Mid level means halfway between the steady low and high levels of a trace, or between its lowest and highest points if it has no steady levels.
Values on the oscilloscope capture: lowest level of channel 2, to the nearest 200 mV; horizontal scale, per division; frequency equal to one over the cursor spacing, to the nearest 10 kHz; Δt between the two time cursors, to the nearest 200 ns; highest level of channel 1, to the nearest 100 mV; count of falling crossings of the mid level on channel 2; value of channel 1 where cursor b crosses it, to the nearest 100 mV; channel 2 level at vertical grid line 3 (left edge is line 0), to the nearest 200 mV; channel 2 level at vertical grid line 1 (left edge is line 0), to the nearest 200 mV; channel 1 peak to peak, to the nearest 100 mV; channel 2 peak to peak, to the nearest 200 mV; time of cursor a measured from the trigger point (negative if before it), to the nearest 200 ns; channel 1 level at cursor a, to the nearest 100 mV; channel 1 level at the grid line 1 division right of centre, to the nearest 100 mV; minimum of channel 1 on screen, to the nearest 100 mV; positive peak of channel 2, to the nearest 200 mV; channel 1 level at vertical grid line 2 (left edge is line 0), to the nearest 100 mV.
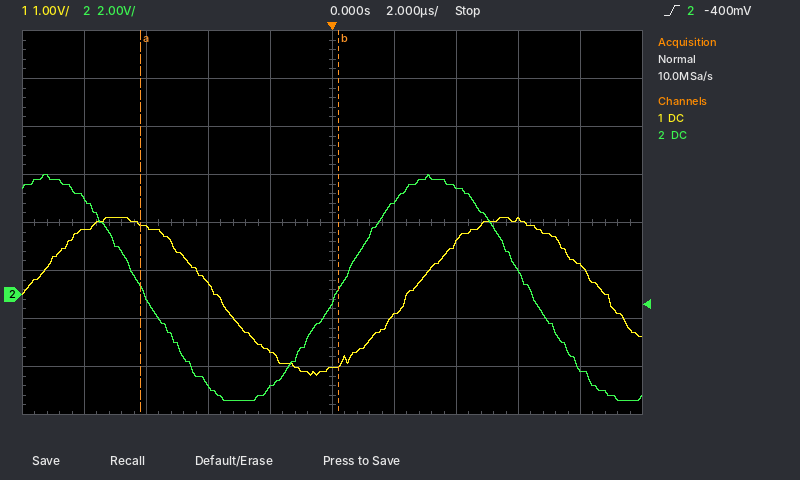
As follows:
-4.4 V
2 µs
160 kHz
6.4 µs
1.6 V
2
-1.5 V
-3.8 V
4.0 V
3.3 V
9.4 V
-6.2 µs
1.5 V
-400 mV
-1.7 V
5.0 V
1.4 V
